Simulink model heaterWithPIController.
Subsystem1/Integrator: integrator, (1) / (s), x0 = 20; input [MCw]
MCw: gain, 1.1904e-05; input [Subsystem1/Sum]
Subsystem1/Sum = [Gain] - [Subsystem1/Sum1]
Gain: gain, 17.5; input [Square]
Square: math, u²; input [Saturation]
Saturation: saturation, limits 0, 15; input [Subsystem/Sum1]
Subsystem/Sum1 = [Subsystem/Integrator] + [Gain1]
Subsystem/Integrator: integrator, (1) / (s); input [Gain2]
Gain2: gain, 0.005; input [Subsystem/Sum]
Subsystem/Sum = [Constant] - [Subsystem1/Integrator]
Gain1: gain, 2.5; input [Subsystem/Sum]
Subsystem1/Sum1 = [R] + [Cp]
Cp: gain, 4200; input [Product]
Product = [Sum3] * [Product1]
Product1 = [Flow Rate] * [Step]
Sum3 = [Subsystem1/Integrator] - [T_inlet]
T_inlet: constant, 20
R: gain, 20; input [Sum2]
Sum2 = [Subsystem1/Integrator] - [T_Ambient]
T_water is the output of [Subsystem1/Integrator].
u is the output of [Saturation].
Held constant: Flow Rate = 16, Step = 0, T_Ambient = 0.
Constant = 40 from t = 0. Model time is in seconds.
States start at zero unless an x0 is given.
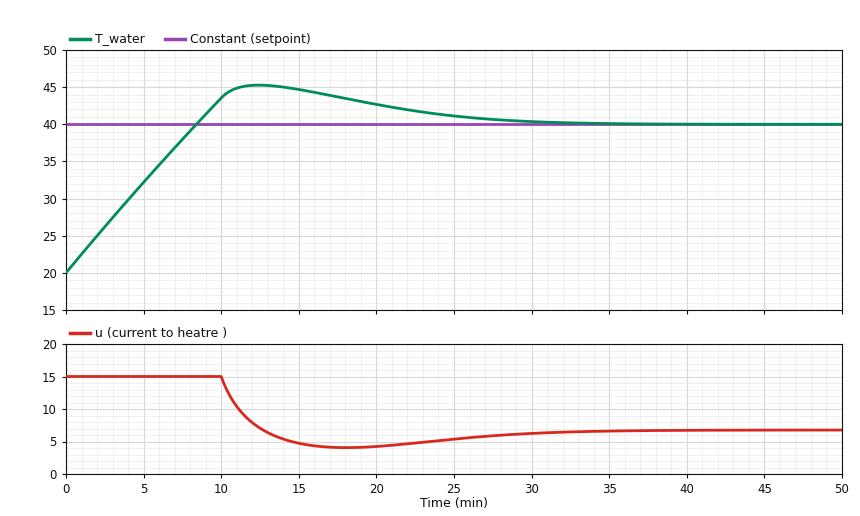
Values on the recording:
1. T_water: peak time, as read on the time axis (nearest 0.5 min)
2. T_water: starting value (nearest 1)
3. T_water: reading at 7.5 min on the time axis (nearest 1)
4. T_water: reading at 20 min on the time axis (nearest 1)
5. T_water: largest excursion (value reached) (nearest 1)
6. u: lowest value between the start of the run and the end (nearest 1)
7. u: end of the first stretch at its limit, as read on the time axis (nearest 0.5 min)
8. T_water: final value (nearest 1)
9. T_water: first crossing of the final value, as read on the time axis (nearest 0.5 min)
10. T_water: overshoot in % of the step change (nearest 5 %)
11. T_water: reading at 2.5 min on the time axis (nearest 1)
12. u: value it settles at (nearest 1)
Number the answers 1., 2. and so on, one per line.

1. 12.5 min
2. 20
3. 38
4. 43
5. 45
6. 4
7. 10.0 min
8. 40
9. 8.5 min
10. 25 %
11. 26
12. 7
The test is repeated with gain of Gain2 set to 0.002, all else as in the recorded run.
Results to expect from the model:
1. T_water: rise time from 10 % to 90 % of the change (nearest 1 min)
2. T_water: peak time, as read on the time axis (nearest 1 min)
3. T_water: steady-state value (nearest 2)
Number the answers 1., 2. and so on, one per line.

1. 7 min
2. 15 min
3. 40
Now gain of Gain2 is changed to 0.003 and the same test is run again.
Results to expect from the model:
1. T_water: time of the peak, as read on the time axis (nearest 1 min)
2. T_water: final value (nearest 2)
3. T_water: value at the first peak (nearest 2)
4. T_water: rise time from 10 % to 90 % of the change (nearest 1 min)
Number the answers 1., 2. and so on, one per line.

1. 13 min
2. 40
3. 42
4. 7 min
